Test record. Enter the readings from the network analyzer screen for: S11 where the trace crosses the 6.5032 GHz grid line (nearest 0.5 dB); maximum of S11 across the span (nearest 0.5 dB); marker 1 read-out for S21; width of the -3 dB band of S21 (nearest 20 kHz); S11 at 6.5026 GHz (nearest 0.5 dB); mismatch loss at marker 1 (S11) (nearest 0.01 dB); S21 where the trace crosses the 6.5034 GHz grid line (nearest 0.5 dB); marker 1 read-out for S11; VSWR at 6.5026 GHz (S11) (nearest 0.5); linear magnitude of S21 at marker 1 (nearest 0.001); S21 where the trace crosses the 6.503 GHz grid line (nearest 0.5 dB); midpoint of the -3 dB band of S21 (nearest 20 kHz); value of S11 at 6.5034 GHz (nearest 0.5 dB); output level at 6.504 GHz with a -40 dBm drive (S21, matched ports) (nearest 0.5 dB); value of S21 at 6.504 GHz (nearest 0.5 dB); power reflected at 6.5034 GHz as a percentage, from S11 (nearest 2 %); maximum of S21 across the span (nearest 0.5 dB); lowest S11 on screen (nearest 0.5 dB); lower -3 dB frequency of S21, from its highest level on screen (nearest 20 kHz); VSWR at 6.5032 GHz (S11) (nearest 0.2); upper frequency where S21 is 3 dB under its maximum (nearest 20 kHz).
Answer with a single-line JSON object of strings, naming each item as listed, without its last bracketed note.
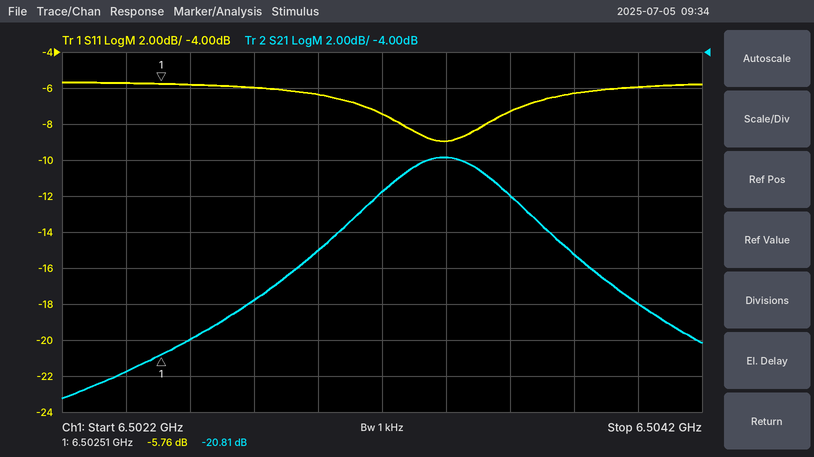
{"S11 where the trace crosses the 6.5032 GHz grid line": "-7.5 dB", "maximum of S11 across the span": "-5.5 dB", "marker 1 read-out for S21": "-20.81 dB", "width of the -3 dB band of S21": "520 kHz", "S11 at 6.5026 GHz": "-6.0 dB", "mismatch loss at marker 1 (S11)": "1.34 dB", "S21 where the trace crosses the 6.5034 GHz grid line": "-10.0 dB", "marker 1 read-out for S11": "-5.76 dB", "VSWR at 6.5026 GHz (S11)": "3.0", "linear magnitude of S21 at marker 1": "0.091", "S21 where the trace crosses the 6.503 GHz grid line": "-15.0 dB", "midpoint of the -3 dB band of S21": "6.50340 GHz", "value of S11 at 6.5034 GHz": "-9.0 dB", "output level at 6.504 GHz with a -40 dBm drive (S21, matched ports)": "-58.0 dBm", "value of S21 at 6.504 GHz": "-18.0 dB", "power reflected at 6.5034 GHz as a percentage, from S11": "12 %", "maximum of S21 across the span": "-10.0 dB", "lowest S11 on screen": "-9.0 dB", "lower -3 dB frequency of S21, from its highest level on screen": "6.50314 GHz", "VSWR at 6.5032 GHz (S11)": "2.4", "upper frequency where S21 is 3 dB under its maximum": "6.50366 GHz"}
